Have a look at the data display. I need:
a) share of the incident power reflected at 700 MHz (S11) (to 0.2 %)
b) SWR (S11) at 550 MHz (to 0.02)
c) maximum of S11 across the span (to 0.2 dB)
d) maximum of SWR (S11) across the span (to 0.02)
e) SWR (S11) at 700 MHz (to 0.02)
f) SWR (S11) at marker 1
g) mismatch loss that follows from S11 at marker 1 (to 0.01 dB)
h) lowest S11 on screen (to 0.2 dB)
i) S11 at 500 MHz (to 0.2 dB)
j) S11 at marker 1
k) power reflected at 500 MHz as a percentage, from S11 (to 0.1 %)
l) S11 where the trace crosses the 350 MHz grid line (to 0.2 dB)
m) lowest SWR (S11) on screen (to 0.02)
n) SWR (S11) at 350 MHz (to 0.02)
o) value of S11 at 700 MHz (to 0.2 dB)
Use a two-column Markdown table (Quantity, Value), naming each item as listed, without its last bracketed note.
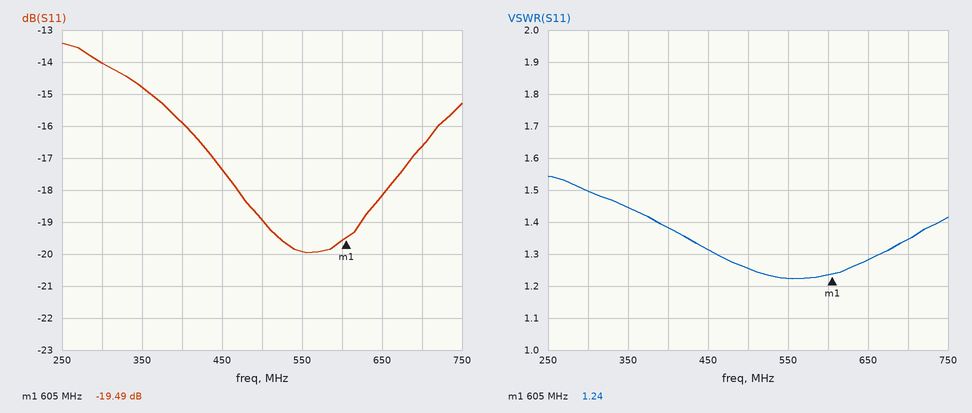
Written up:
| Quantity | Value |
|---|---|
| share of the incident power reflected at 700 MHz (S11) | 2.2 % |
| SWR (S11) at 550 MHz | 1.22 |
| maximum of S11 across the span | -13.4 dB |
| maximum of SWR (S11) across the span | 1.54 |
| SWR (S11) at 700 MHz | 1.34 |
| SWR (S11) at marker 1 | 1.24 |
| mismatch loss that follows from S11 at marker 1 | 0.05 dB |
| lowest S11 on screen | -20.0 dB |
| S11 at 500 MHz | -19.0 dB |
| S11 at marker 1 | -19.49 dB |
| power reflected at 500 MHz as a percentage, from S11 | 1.3 % |
| S11 where the trace crosses the 350 MHz grid line | -14.8 dB |
| lowest SWR (S11) on screen | 1.22 |
| SWR (S11) at 350 MHz | 1.44 |
| value of S11 at 700 MHz | -16.6 dB |
